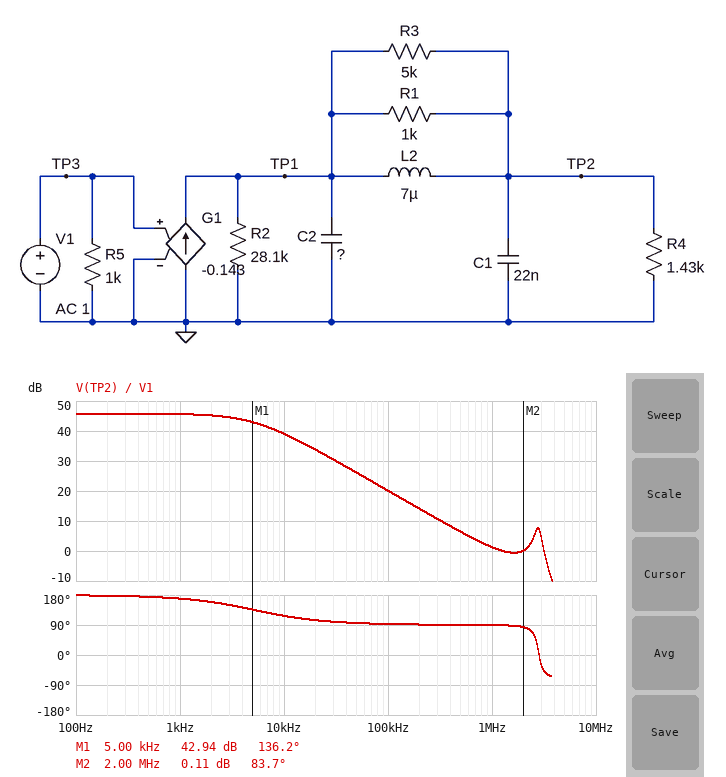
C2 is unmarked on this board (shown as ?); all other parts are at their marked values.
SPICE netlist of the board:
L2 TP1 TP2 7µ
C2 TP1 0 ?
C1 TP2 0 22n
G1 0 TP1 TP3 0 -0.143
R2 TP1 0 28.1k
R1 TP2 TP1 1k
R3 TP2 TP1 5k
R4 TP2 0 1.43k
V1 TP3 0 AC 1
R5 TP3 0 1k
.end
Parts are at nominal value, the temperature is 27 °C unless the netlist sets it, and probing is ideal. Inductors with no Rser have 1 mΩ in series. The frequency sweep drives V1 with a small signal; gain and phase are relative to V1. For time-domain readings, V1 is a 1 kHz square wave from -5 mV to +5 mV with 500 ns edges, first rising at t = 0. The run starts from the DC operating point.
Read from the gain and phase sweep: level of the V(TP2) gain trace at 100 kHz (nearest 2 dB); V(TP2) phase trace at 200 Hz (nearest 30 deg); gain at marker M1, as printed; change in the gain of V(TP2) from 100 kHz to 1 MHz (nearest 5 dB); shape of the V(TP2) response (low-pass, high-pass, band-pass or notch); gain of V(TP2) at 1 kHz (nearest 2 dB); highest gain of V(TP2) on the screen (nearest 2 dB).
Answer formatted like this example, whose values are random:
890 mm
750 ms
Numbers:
20 dB
180 deg
42.94 dB
-20 dB
low-pass
46 dB
46 dB
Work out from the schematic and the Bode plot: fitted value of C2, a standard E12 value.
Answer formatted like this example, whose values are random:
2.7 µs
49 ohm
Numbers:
470 pF
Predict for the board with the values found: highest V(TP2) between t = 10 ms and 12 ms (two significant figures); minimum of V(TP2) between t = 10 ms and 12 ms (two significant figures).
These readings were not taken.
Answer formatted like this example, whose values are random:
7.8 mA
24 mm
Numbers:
970 mV
-970 mV
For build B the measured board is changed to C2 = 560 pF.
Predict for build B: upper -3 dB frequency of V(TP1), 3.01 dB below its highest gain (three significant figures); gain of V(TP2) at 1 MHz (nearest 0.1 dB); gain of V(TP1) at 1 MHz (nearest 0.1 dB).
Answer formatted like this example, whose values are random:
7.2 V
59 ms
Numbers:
5.18 kHz
1.5 dB
15.6 dB
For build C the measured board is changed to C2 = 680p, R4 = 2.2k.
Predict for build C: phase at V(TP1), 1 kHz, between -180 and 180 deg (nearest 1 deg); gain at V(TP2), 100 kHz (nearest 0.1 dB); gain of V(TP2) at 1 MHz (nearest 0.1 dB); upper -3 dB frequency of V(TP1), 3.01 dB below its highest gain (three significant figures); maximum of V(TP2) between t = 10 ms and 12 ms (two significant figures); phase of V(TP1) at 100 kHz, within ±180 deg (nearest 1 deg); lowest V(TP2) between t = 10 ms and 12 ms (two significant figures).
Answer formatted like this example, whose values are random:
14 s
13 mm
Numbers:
164 deg
20.0 dB
1.8 dB
3.44 kHz
1.5 V
92 deg
-1.5 V
